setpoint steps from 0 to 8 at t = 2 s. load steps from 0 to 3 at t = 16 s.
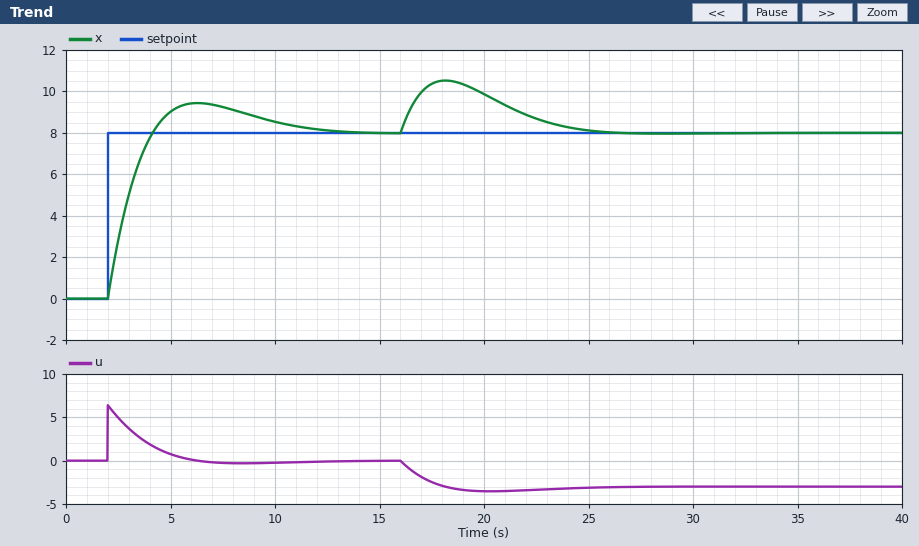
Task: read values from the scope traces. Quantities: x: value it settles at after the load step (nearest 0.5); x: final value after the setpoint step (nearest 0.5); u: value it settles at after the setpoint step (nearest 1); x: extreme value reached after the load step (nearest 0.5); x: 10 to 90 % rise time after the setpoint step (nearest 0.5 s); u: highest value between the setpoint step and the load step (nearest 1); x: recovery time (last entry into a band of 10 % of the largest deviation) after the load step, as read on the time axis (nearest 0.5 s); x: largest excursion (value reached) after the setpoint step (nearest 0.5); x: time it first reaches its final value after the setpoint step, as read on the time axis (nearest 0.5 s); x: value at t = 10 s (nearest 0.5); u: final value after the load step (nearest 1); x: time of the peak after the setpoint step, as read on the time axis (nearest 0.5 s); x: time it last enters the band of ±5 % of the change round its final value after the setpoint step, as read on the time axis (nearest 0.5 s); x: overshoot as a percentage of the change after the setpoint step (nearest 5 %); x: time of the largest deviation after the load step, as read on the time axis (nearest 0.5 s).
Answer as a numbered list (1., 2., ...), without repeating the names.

1. 8.0
2. 8.0
3. 0
4. 10.5
5. 1.5 s
6. 6
7. 24.0 s
8. 9.5
9. 4.0 s
10. 8.5
11. -3
12. 6.5 s
13. 10.5 s
14. 20 %
15. 18.0 s
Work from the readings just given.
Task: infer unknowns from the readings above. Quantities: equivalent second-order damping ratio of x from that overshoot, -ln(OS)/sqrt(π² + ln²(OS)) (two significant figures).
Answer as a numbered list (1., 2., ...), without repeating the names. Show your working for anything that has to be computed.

1. ln(0.2) = -1.609; 1.609 / sqrt(9.870 + 2.590) = 0.46
